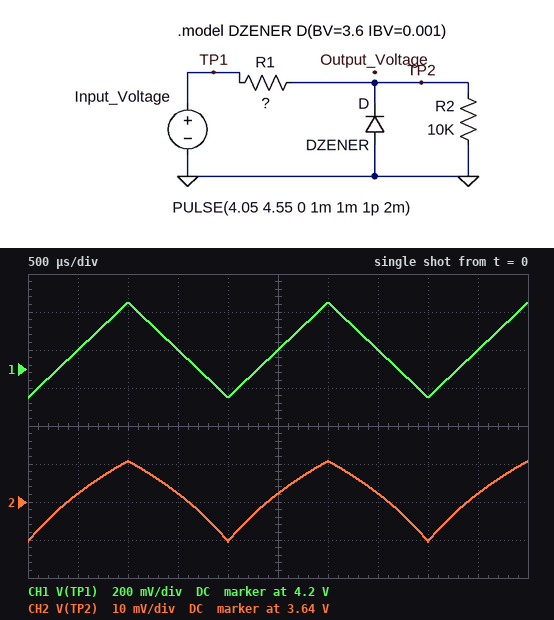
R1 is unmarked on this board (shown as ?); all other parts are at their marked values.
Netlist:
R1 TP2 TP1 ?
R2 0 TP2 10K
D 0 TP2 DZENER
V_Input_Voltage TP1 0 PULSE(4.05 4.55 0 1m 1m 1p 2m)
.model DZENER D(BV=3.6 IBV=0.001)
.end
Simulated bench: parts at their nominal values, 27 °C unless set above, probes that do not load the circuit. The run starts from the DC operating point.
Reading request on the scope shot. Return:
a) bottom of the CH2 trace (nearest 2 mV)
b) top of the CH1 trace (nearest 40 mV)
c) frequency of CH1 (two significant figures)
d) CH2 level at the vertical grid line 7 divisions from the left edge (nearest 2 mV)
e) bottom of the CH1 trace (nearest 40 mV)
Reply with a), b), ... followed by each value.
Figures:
a) 3.630 V
b) 4.56 V
c) 500 Hz
d) 3.642 V
e) 4.04 V
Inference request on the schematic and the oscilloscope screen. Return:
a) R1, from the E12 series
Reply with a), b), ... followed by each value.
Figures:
a) 120 Ω
